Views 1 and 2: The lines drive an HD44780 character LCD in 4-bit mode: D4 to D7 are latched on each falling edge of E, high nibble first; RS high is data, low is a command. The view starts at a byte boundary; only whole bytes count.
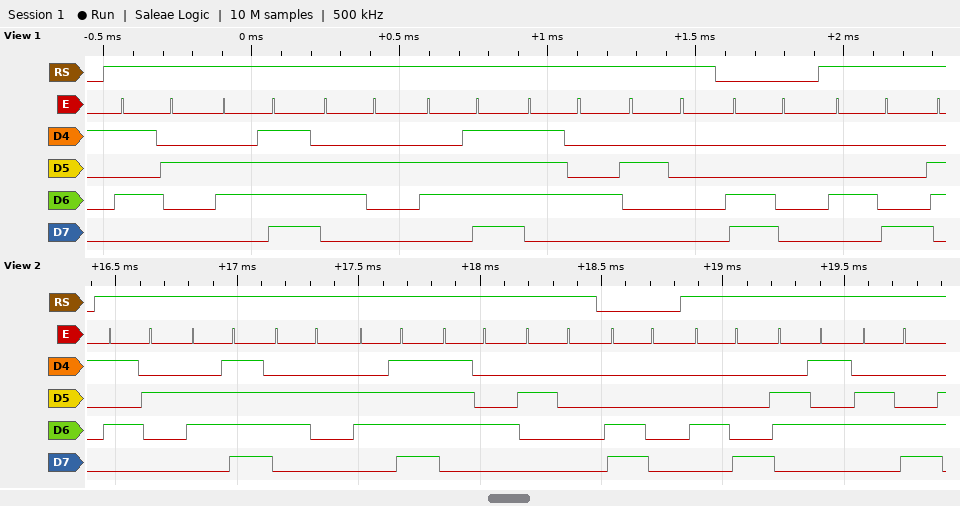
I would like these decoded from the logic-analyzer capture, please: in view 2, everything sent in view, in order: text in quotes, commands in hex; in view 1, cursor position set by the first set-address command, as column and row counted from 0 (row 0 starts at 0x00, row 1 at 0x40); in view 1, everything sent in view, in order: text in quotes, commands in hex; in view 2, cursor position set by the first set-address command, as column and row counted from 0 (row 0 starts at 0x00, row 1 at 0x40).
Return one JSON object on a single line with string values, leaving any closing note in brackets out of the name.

{"in view 2, everything sent in view, in order: text in quotes, commands in hex": "\"Robot \" 0xC0 \"Hel\"", "in view 1, cursor position set by the first set-address command, as column and row counted from 0": "column 0, row 1", "in view 1, everything sent in view, in order: text in quotes, commands in hex": "\"Robot \" 0xC0 \"H\"", "in view 2, cursor position set by the first set-address command, as column and row counted from 0": "column 0, row 1"}
